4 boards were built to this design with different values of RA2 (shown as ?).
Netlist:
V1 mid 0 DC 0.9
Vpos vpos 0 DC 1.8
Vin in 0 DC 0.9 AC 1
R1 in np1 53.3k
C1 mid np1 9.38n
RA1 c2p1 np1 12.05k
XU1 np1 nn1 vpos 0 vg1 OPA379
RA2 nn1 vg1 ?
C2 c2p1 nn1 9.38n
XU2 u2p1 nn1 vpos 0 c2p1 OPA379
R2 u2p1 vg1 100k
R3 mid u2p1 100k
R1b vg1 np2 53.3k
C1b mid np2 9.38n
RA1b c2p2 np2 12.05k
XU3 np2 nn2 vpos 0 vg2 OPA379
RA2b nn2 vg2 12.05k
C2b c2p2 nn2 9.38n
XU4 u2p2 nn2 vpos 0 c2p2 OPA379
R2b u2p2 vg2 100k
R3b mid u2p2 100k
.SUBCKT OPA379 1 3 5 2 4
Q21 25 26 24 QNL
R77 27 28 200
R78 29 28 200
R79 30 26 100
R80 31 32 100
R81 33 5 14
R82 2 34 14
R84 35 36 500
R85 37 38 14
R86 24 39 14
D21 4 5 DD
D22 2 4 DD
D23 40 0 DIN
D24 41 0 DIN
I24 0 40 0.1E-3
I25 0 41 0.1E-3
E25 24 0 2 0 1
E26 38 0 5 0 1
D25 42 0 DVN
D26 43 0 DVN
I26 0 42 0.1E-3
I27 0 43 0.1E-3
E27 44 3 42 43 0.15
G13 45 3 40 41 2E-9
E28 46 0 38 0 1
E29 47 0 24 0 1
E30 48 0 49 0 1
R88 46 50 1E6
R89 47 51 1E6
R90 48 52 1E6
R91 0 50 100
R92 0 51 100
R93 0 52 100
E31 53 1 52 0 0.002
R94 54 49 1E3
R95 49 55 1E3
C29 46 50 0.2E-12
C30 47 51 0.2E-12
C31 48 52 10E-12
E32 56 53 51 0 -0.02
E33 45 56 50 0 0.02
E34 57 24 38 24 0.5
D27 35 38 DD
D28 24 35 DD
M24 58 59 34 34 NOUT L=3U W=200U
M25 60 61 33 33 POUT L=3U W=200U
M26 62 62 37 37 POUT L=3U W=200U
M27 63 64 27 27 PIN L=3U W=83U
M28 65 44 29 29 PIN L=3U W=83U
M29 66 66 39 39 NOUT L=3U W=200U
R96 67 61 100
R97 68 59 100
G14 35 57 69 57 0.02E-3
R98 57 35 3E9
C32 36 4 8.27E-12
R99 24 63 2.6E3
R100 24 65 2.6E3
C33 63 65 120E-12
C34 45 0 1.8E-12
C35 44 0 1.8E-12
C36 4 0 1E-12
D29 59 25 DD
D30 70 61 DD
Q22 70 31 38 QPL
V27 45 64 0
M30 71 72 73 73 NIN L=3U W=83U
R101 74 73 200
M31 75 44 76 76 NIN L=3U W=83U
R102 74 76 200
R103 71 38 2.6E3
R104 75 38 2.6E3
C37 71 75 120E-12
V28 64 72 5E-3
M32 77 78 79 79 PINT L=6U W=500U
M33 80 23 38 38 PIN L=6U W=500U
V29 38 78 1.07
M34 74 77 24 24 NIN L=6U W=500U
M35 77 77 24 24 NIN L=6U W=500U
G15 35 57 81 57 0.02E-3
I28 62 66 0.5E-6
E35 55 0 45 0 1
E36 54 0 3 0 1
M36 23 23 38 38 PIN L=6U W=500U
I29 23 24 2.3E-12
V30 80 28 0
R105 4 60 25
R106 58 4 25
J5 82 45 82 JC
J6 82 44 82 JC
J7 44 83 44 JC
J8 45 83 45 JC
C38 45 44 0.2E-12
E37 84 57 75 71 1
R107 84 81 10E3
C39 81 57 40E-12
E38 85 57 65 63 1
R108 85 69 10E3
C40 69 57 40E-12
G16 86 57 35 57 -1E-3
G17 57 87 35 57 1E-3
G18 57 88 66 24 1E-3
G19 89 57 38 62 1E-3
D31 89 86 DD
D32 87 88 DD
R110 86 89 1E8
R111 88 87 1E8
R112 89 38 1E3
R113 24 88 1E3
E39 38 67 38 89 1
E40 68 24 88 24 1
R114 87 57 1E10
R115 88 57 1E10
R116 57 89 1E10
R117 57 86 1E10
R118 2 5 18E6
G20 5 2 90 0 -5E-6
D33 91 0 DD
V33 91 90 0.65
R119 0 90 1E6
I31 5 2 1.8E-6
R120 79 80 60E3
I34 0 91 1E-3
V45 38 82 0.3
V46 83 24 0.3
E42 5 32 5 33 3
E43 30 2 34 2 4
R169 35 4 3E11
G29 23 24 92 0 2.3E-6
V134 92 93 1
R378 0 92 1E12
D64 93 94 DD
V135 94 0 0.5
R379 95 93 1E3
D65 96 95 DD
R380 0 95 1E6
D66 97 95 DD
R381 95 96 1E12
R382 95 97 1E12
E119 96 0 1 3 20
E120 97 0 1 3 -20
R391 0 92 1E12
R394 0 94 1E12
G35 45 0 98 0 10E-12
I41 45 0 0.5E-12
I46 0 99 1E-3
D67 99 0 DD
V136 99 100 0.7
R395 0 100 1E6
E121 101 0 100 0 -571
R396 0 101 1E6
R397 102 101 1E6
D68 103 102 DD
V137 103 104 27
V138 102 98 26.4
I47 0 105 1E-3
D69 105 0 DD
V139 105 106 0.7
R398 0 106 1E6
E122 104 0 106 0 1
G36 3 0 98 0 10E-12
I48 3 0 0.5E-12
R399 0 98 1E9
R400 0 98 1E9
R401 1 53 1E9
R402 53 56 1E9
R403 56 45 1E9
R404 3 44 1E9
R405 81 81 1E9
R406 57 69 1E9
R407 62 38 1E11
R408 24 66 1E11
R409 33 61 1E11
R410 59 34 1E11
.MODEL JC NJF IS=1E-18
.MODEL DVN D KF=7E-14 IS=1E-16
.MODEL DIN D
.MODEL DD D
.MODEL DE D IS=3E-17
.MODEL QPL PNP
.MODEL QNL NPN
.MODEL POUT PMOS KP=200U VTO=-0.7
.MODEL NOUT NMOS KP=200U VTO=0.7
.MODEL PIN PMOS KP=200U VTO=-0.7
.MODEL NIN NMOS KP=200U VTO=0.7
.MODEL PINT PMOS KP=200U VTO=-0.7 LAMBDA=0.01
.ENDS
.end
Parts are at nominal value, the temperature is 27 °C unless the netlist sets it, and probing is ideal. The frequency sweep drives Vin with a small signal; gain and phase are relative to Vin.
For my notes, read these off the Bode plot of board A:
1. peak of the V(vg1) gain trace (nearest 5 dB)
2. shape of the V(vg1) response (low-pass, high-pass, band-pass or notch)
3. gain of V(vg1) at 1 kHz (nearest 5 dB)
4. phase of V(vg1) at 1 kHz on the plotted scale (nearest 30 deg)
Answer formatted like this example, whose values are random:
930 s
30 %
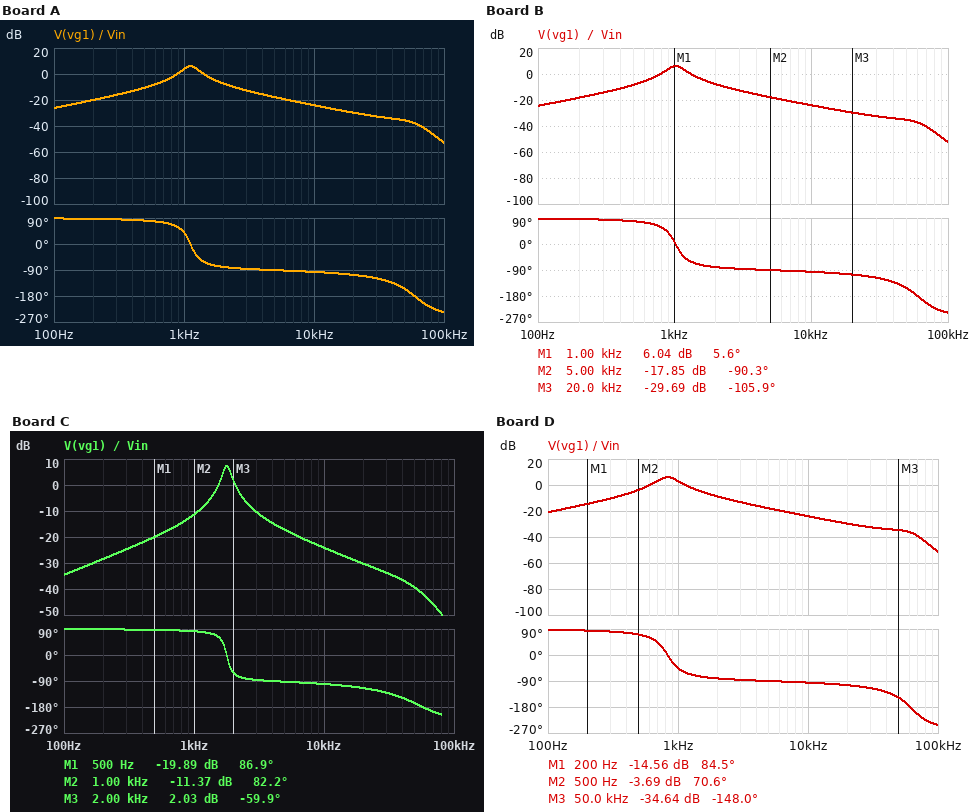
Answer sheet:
5 dB
band-pass
5 dB
30 deg
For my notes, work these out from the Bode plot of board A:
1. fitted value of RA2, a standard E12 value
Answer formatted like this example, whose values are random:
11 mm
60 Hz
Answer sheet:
18 kΩ
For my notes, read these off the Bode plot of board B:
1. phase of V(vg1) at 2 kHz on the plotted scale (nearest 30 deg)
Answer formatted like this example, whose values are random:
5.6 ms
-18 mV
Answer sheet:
-90 deg
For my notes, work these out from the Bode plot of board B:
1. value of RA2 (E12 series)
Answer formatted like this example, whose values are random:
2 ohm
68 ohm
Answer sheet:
22 kΩ
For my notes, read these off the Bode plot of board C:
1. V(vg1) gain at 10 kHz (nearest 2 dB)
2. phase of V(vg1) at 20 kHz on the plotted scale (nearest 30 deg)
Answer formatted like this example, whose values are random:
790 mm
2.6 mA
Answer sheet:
-24 dB
-120 deg
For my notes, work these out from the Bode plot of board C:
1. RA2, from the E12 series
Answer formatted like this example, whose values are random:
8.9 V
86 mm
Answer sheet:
6.8 kΩ
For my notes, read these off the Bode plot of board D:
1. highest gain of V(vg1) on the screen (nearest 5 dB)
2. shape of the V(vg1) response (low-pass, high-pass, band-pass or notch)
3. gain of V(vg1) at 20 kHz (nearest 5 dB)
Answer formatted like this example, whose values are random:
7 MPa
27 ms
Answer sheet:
5 dB
band-pass
-30 dB
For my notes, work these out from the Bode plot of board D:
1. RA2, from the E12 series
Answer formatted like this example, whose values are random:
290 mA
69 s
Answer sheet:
33 kΩ
